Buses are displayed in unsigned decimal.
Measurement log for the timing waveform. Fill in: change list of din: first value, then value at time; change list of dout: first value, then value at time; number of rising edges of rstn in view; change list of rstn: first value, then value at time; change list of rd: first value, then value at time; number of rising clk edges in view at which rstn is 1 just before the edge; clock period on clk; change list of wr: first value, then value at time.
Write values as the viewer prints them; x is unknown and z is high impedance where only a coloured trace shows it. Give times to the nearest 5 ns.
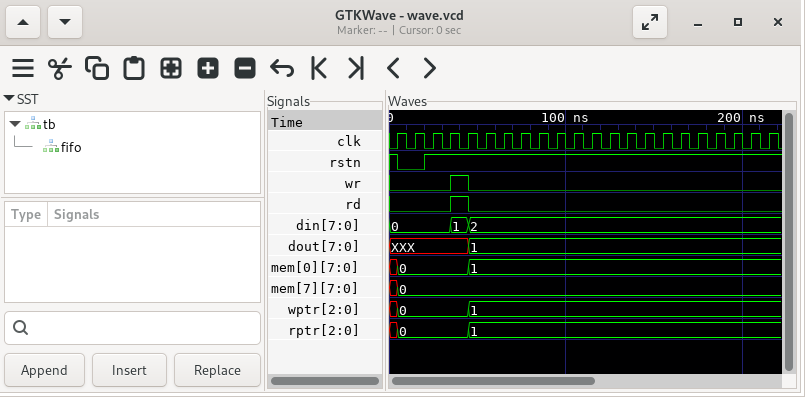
0, 1 at 35 ns, 2 at 45 ns
XXX, 1 at 45 ns
1
1, 0 at 5 ns, 1 at 20 ns
0, 1 at 35 ns, 0 at 45 ns
21
10 ns
0, 1 at 35 ns, 0 at 45 ns
